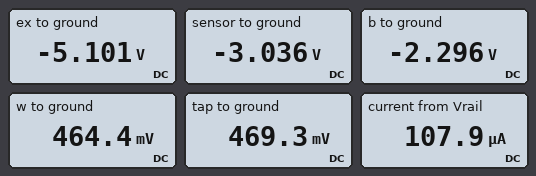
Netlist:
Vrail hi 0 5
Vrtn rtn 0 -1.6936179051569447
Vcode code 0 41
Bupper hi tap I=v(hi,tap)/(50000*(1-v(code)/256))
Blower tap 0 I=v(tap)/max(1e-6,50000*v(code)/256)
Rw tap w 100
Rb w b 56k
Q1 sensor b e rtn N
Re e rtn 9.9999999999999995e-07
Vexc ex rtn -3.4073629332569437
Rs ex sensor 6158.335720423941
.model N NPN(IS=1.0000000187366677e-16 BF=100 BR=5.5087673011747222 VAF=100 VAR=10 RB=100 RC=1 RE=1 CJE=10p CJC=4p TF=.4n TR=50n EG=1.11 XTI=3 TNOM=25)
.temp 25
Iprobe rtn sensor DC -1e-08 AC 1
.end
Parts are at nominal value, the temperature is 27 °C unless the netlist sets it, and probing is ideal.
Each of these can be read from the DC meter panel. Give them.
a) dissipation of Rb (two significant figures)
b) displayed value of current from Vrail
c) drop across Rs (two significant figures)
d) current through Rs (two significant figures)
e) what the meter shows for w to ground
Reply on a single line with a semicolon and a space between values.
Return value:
140 µW; 107.9 µA; 2.1 V; 340 µA; 464.4 mV
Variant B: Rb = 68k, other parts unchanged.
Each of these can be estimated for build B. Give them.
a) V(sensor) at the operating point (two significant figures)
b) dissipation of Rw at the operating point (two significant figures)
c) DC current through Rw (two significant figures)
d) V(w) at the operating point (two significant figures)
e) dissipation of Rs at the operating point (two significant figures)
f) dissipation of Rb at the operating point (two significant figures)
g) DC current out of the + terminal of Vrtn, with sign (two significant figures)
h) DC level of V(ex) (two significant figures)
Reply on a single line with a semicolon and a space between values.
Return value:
-3.2 V; 190 nW; 44 µA; 500 mV; 570 µW; 130 µW; -44 µA; -5.1 V
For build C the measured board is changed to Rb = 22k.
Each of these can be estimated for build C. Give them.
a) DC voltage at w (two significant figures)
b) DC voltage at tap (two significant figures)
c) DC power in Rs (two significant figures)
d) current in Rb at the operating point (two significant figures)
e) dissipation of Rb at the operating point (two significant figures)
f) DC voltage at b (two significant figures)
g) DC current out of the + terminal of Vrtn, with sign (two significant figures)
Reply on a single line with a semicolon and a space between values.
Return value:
280 mV; 290 mV; 1.4 mW; 76 µA; 130 µW; -1.4 V; -76 µA
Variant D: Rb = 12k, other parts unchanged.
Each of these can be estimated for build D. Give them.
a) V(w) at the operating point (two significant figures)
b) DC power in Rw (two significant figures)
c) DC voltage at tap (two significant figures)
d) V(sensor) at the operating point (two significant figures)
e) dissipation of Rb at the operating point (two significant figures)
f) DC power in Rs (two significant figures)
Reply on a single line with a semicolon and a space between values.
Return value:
150 mV; 910 nW; 160 mV; -1.8 V; 110 µW; 1.8 mW
